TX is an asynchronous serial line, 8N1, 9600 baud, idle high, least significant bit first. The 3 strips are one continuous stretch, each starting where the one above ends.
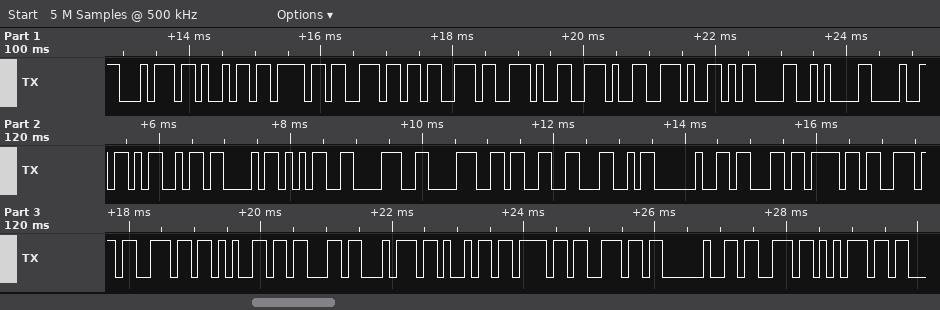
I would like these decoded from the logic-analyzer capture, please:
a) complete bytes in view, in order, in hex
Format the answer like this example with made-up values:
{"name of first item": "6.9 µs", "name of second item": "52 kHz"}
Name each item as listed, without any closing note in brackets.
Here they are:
{"complete bytes in view, in order, in hex": "74 69 6F 6E 73 2E 2E 2E 0D 0A 48 4D 43 35 38 38 33 4C 20 63 6F 6E 6E 65 63 74 69 6F 6E 20 73 75"}
